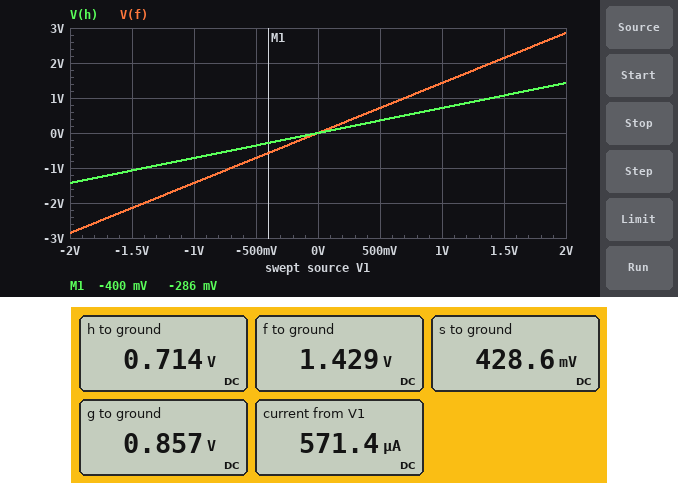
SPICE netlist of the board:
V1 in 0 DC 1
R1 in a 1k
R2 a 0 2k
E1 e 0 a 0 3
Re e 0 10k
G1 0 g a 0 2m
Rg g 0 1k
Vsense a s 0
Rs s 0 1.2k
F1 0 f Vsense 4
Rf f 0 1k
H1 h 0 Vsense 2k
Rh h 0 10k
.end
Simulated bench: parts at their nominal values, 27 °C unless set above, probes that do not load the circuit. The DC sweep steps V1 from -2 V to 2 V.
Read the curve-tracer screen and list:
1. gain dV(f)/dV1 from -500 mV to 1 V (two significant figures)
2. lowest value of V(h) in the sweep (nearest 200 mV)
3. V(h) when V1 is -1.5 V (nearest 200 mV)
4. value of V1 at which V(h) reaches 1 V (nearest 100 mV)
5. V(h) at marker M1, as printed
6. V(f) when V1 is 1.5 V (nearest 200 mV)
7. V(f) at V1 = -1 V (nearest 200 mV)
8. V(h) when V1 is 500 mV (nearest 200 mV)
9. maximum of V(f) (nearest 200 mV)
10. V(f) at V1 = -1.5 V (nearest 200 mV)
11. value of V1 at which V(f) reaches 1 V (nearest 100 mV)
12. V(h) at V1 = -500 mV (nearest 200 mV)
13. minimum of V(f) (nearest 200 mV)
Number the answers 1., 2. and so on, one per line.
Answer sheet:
1. 1.4 V/V
2. -1.4 V
3. -1.0 V
4. 1.4 V
5. -286 mV
6. 2.2 V
7. -1.4 V
8. 400 mV
9. 2.8 V
10. -2.2 V
11. 700 mV
12. -400 mV
13. -2.8 V
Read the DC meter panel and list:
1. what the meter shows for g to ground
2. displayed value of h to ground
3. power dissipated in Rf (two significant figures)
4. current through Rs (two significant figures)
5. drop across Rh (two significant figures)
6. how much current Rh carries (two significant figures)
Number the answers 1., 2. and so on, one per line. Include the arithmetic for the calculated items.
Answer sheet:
1. 0.857 V
2. 0.714 V
3. (1.429 V)^2 / 1 kΩ = 2.0 mW
4. (428.6 mV) / 1.2 kΩ = 360 µA
5. 714 mV = 710 mV
6. (714 mV) / 10 kΩ = 71 µA
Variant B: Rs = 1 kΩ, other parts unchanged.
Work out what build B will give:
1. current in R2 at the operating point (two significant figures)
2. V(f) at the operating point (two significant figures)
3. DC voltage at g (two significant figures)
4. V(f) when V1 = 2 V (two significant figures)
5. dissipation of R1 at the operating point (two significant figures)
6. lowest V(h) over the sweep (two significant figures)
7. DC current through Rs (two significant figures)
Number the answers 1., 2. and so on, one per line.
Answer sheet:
1. 200 µA
2. 1.6 V
3. 800 mV
4. 3.2 V
5. 360 µW
6. -1.6 V
7. 400 µA
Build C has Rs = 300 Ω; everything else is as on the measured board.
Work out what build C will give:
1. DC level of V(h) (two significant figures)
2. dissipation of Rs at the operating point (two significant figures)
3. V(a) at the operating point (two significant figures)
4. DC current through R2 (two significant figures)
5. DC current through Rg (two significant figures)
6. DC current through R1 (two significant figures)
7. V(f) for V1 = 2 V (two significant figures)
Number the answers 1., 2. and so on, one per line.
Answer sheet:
1. 1.4 V
2. 140 µW
3. 210 mV
4. 100 µA
5. 410 µA
6. 790 µA
7. 5.5 V
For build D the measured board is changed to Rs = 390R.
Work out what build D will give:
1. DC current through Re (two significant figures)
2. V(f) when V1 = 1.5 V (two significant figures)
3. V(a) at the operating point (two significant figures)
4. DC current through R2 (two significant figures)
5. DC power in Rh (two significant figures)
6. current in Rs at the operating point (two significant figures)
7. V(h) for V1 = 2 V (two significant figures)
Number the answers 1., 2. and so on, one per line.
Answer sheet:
1. 74 µA
2. 3.8 V
3. 250 mV
4. 120 µA
5. 160 µW
6. 630 µA
7. 2.5 V
